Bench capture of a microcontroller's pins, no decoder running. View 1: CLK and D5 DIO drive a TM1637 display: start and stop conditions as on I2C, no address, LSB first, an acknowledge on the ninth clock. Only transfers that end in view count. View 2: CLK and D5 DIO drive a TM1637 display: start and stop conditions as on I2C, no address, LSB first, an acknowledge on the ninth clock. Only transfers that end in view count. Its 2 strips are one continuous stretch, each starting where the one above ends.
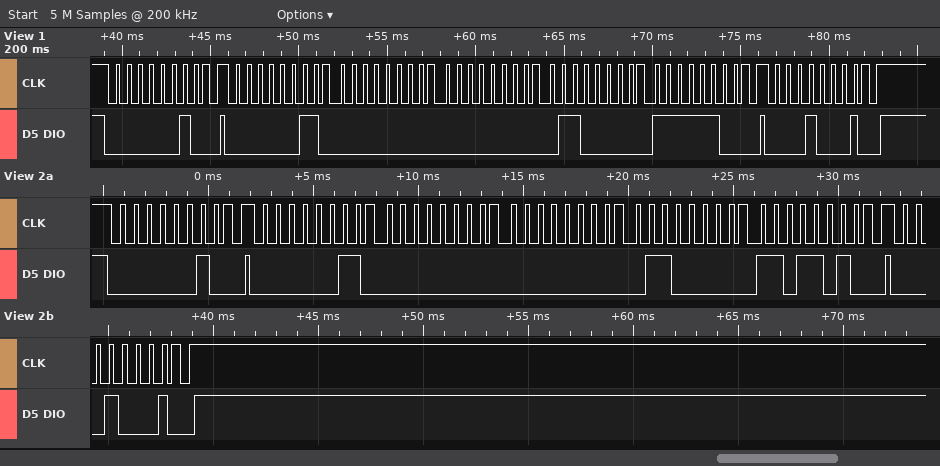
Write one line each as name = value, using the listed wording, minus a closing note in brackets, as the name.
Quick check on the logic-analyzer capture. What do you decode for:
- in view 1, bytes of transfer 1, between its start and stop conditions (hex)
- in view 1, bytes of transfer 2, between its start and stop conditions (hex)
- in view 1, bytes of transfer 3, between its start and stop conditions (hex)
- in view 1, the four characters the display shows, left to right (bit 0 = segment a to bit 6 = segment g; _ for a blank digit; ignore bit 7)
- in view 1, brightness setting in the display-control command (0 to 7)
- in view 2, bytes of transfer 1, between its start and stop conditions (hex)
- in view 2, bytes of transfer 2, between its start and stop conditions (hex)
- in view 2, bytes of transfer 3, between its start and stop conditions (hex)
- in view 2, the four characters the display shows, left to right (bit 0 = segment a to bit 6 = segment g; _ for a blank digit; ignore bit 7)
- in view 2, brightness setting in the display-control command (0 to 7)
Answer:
in view 1, bytes of transfer 1, between its start and stop conditions = 40
in view 1, bytes of transfer 2, between its start and stop conditions = C0 00 00 06 3F
in view 1, bytes of transfer 3, between its start and stop conditions = 88
in view 1, the four characters the display shows, left to right = __10
in view 1, brightness setting in the display-control command = 0
in view 2, bytes of transfer 1, between its start and stop conditions = 40
in view 2, bytes of transfer 2, between its start and stop conditions = C0 00 00 06 5B
in view 2, bytes of transfer 3, between its start and stop conditions = 88
in view 2, the four characters the display shows, left to right = __12
in view 2, brightness setting in the display-control command = 0
